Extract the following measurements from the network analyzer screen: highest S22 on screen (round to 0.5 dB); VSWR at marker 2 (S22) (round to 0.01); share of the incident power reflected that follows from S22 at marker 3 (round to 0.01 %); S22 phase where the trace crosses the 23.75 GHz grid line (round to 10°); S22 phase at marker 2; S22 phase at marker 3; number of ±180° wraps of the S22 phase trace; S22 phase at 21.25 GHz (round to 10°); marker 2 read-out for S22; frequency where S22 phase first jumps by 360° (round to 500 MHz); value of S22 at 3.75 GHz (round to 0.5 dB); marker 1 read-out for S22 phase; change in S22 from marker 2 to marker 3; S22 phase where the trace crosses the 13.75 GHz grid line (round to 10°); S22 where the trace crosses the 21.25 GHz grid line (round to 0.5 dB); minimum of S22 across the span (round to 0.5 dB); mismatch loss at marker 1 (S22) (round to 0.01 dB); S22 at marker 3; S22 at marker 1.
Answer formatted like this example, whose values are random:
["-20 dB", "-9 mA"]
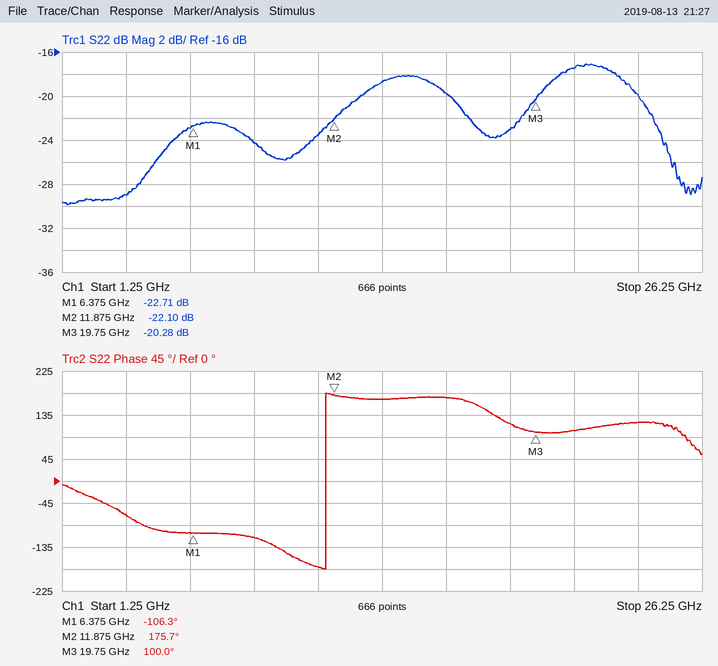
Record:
["-17.0 dB", "1.17", "0.94 %", "120°", "175.7°", "100.0°", "1", "100°", "-22.10 dB", "11.5 GHz", "-29.0 dB", "-106.3°", "1.82 dB", "170°", "-17.5 dB", "-30.0 dB", "0.02 dB", "-20.28 dB", "-22.71 dB"]
